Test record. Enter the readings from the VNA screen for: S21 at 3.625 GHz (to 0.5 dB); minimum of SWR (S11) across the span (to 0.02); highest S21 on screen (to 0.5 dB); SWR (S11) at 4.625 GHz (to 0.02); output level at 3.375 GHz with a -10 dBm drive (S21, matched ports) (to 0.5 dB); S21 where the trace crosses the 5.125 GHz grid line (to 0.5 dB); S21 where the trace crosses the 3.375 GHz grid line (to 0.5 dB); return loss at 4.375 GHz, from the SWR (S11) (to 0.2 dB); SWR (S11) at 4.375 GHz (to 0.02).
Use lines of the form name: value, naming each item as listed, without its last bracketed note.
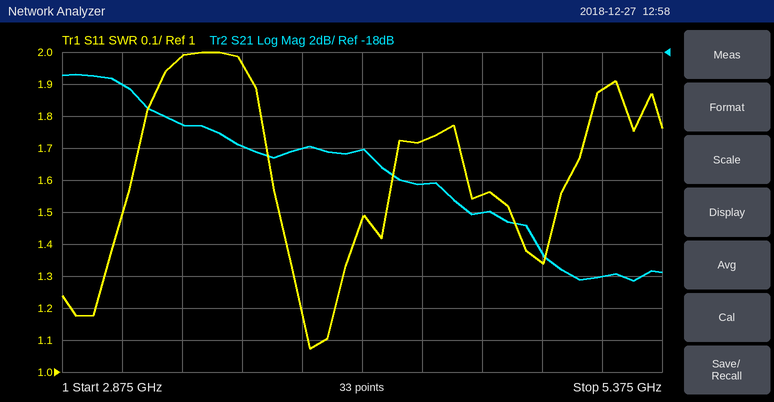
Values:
S21 at 3.625 GHz: -24.0 dB
minimum of SWR (S11) across the span: 1.08
highest S21 on screen: -19.5 dB
SWR (S11) at 4.625 GHz: 1.56
output level at 3.375 GHz with a -10 dBm drive (S21, matched ports): -32.5 dBm
S21 where the trace crosses the 5.125 GHz grid line: -32.0 dB
S21 where the trace crosses the 3.375 GHz grid line: -22.5 dB
return loss at 4.375 GHz, from the SWR (S11): 11.6 dB
SWR (S11) at 4.375 GHz: 1.72
